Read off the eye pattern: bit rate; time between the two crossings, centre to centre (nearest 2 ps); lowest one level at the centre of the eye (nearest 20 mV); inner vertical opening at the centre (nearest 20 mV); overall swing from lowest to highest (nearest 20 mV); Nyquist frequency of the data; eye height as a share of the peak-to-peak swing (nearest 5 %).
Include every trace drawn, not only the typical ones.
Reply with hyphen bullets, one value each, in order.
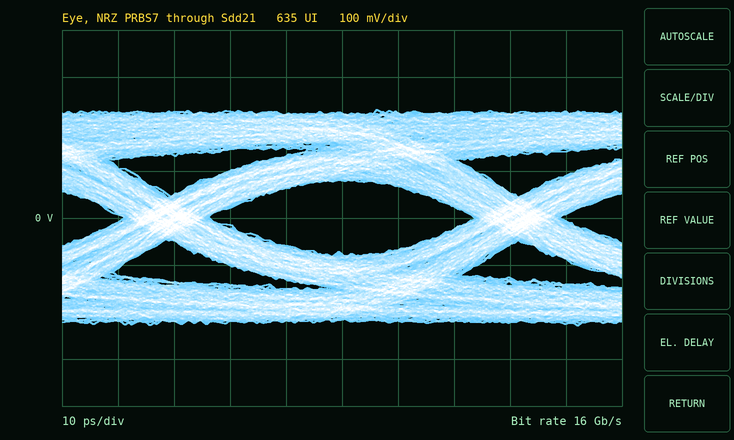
- 16 Gb/s
- 62 ps
- 80 mV
- 160 mV
- 460 mV
- 8 GHz
- 35 %
